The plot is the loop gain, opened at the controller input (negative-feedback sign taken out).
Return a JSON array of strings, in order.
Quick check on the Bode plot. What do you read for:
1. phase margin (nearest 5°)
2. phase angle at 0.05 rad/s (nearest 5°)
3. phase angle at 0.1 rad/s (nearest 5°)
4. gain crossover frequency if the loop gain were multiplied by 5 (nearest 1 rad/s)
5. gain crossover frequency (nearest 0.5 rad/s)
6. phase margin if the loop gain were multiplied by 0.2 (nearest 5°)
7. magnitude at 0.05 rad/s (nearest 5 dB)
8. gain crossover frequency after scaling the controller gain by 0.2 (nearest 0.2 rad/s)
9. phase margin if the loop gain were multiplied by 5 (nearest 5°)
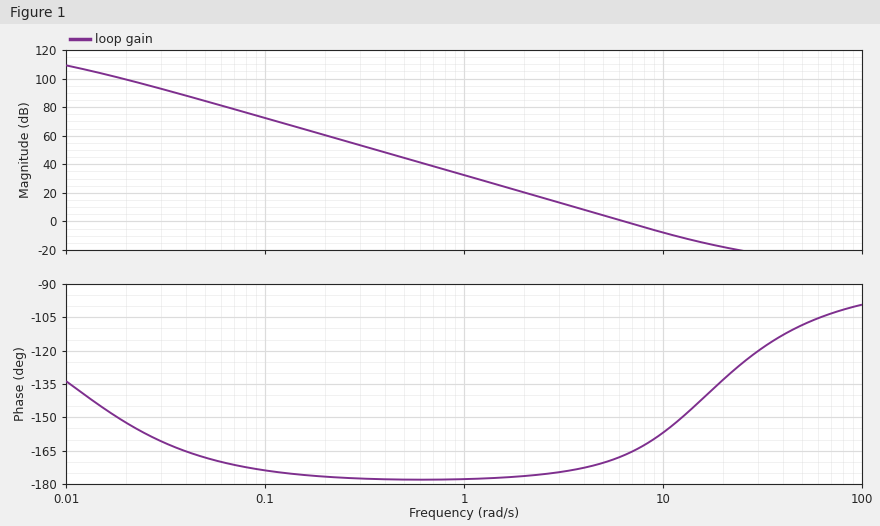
["15°", "-170°", "-175°", "15 rad/s", "6.5 rad/s", "5°", "85 dB", "2.8 rad/s", "35°"]
